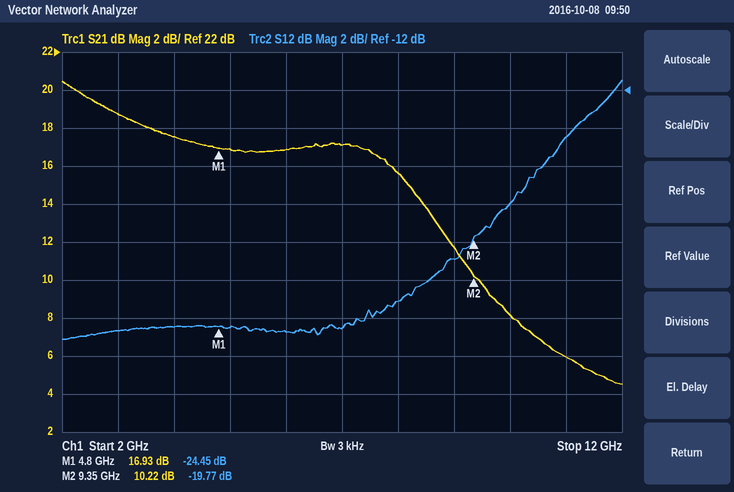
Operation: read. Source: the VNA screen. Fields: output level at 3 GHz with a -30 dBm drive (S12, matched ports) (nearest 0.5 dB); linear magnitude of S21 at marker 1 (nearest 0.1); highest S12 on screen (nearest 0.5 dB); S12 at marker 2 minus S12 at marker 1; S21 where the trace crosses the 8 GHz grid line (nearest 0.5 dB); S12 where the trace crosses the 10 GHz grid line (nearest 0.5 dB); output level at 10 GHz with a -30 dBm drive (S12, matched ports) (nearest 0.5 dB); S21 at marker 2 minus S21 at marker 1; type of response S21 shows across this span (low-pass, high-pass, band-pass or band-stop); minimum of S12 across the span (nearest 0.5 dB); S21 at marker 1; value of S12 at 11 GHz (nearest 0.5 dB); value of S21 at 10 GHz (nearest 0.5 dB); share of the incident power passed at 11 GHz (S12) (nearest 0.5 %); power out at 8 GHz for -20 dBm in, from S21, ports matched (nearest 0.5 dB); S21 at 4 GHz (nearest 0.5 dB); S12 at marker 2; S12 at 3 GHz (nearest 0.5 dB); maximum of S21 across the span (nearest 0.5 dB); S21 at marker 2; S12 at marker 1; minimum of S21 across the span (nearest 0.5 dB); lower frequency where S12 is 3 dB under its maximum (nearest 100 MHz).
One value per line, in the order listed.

-54.5 dBm
7.0
-11.5 dB
4.68 dB
15.5 dB
-18.0 dB
-48.0 dBm
-6.71 dB
low-pass
-25.0 dB
16.93 dB
-14.5 dB
8.0 dB
3.5 %
-4.5 dBm
17.5 dB
-19.77 dB
-24.5 dB
20.5 dB
10.22 dB
-24.45 dB
4.5 dB
11.0 GHz
